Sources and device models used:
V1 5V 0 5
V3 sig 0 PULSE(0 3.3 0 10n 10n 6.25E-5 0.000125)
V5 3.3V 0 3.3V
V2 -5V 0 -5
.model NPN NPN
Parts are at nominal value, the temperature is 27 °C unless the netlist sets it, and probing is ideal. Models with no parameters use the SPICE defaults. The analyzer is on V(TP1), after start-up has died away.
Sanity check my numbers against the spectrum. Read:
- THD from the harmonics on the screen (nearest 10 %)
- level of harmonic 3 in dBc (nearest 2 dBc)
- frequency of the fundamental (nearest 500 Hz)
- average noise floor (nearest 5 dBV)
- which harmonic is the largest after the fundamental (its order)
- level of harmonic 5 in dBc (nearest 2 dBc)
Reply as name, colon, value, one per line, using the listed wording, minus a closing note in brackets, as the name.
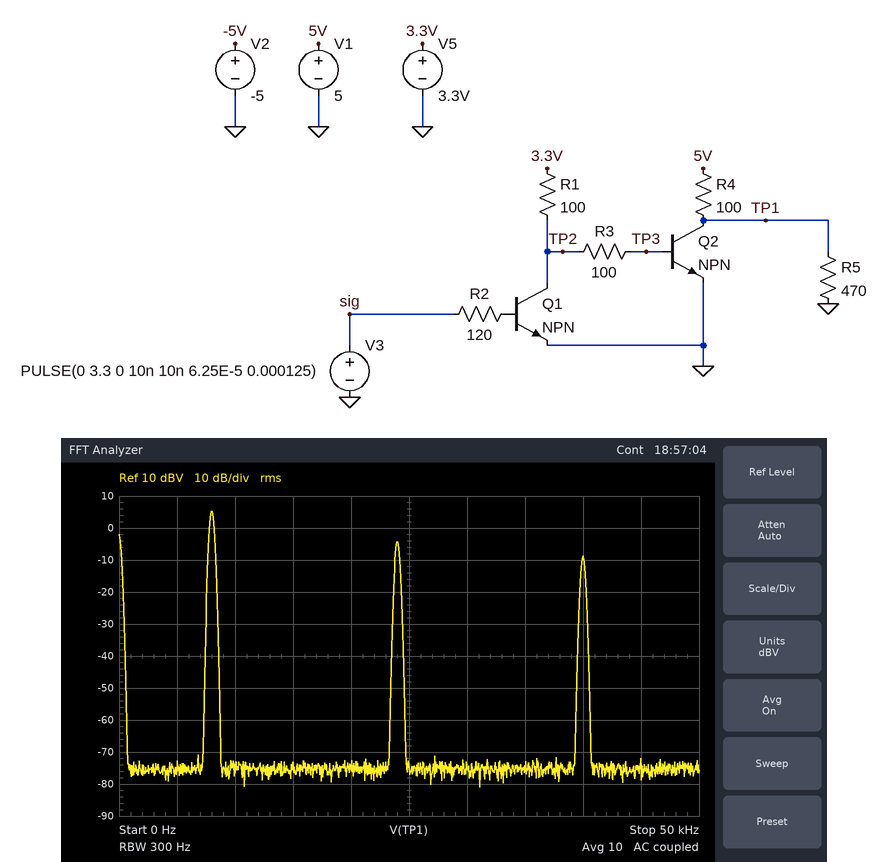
THD from the harmonics on the screen: 40 %
level of harmonic 3 in dBc: -10 dBc
frequency of the fundamental: 8.0 kHz
average noise floor: -75 dBV
which harmonic is the largest after the fundamental: 3
level of harmonic 5 in dBc: -14 dBc
